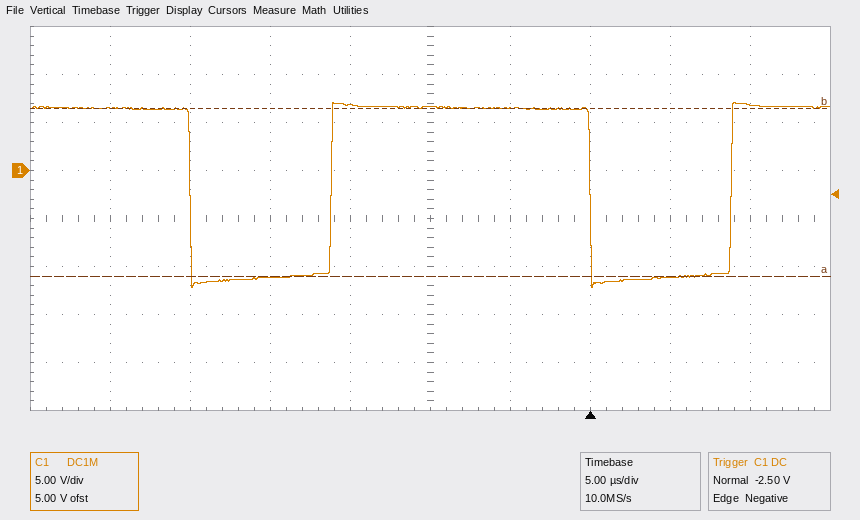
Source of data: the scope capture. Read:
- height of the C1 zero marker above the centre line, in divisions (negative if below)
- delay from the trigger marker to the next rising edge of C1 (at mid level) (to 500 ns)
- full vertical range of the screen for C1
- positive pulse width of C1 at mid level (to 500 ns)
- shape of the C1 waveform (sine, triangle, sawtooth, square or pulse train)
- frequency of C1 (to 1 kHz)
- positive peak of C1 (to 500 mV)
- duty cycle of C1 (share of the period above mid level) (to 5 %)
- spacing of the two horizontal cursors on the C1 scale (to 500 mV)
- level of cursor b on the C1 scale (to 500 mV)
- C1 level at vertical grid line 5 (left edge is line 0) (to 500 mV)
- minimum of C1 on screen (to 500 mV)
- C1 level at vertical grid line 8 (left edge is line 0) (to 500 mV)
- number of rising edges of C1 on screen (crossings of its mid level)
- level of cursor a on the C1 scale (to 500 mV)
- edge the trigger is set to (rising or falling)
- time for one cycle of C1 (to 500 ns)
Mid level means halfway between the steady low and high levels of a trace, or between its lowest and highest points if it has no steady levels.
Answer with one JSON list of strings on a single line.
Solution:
["+1.0 div", "9.0 µs", "40 V", "16.0 µs", "pulse train", "40 kHz", "7.0 V", "65 %", "17.5 V", "6.5 V", "6.5 V", "-12.0 V", "-11.0 V", "2", "-11.0 V", "falling", "25.0 µs"]
